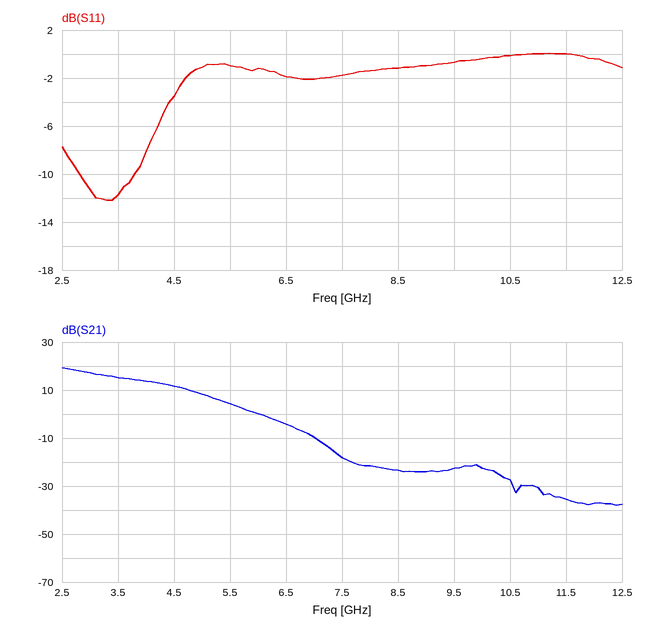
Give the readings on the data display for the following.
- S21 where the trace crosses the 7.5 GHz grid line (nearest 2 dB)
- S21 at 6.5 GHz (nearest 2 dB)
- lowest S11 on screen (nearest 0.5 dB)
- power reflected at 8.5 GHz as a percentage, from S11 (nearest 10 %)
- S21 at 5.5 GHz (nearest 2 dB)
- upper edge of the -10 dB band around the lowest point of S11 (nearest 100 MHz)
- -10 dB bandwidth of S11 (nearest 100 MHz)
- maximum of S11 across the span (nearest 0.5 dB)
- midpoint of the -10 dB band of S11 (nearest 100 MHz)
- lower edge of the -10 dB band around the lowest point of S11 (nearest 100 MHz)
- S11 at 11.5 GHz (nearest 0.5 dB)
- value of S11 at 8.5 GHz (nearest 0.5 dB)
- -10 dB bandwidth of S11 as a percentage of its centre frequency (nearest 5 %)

-18 dB
-4 dB
-12.0 dB
80 %
4 dB
3.8 GHz
1.0 GHz
0.0 dB
3.3 GHz
2.8 GHz
0.0 dB
-1.0 dB
30 %
